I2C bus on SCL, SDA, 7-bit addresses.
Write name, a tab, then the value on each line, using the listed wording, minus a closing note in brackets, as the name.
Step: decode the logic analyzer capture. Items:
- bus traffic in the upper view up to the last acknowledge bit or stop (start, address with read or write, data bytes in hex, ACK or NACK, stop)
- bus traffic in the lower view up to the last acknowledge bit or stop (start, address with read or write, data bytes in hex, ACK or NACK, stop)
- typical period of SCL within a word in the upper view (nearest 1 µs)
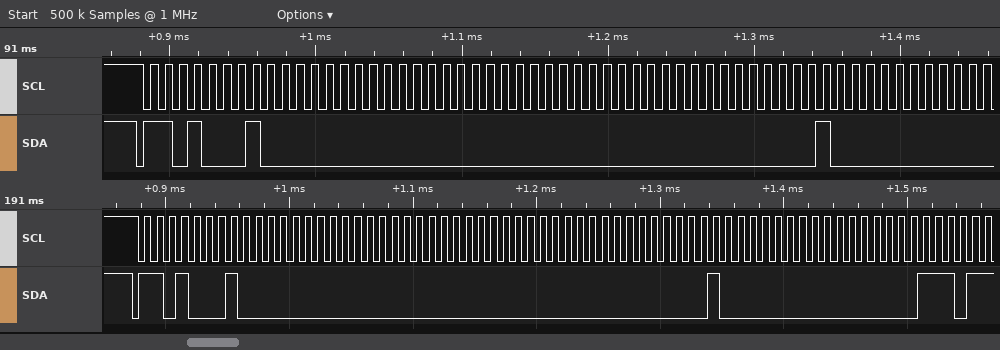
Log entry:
bus traffic in the upper view up to the last acknowledge bit or stop	start, address 68 read ACK, 00 ACK, 00 ACK, 00 ACK, 00 ACK, 40 ACK
bus traffic in the lower view up to the last acknowledge bit or stop	start, address 68 read ACK, 00 ACK, 00 ACK, 00 ACK, 00 ACK, 40 ACK, 00 ACK
typical period of SCL within a word in the upper view	10 µs
